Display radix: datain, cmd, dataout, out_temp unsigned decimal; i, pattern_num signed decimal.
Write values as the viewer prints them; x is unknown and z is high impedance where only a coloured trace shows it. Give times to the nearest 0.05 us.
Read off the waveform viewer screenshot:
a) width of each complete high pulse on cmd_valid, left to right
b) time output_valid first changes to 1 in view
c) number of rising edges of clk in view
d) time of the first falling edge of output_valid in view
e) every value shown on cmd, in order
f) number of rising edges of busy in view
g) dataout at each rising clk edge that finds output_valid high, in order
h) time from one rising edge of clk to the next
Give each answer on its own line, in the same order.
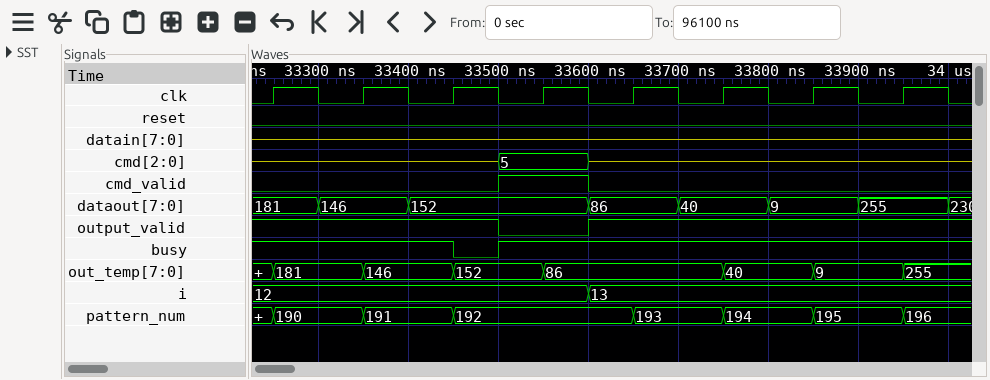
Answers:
0.1 us
33.6 us
8
33.5 us
z, 5, z
1
181, 146, 152, 86, 40, 9, 255
0.1 us
